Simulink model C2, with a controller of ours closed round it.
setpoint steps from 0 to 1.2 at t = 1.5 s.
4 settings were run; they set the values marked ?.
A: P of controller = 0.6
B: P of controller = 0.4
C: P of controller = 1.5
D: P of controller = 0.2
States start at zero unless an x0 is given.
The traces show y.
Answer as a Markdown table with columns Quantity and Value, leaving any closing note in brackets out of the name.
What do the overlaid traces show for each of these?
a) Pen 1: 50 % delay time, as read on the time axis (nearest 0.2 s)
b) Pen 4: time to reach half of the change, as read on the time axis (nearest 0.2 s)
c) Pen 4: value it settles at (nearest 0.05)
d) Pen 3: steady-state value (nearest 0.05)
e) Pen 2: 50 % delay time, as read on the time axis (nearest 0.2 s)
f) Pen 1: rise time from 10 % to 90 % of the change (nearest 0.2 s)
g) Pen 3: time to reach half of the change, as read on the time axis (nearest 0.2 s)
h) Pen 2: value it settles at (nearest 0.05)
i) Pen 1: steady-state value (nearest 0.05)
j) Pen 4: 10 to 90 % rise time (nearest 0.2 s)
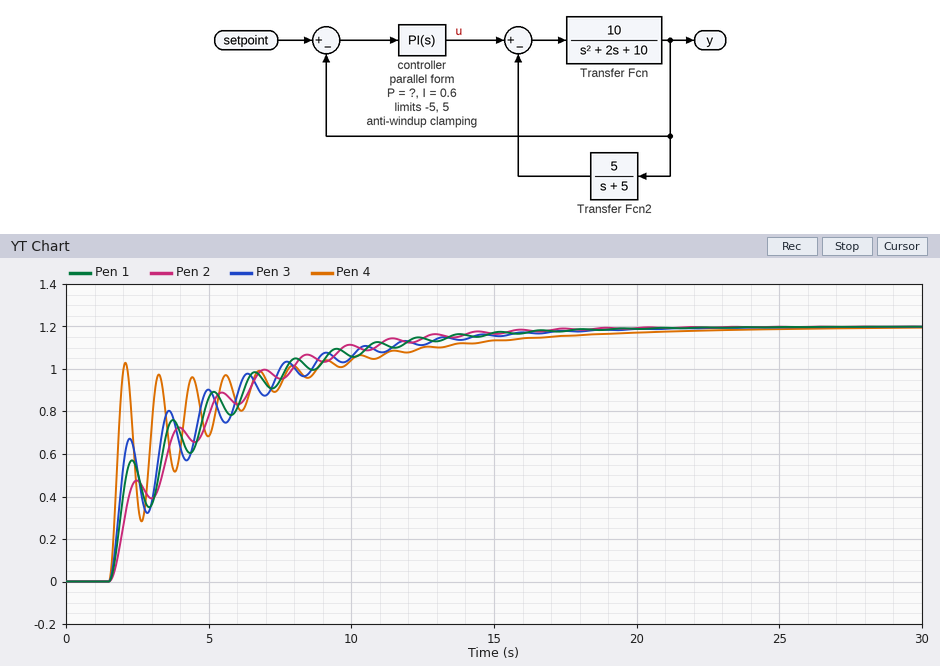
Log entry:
| Quantity | Value |
|---|---|
| Pen 1: 50 % delay time, as read on the time axis | 3.4 s |
| Pen 4: time to reach half of the change, as read on the time axis | 1.8 s |
| Pen 4: value it settles at | 1.20 |
| Pen 3: steady-state value | 1.20 |
| Pen 2: 50 % delay time, as read on the time axis | 3.6 s |
| Pen 1: rise time from 10 % to 90 % of the change | 7.6 s |
| Pen 3: time to reach half of the change, as read on the time axis | 2.0 s |
| Pen 2: value it settles at | 1.20 |
| Pen 1: steady-state value | 1.20 |
| Pen 4: 10 to 90 % rise time | 9.6 s |
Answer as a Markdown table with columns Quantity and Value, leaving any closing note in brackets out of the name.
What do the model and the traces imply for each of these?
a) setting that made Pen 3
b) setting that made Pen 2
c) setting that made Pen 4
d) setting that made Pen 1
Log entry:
| Quantity | Value |
|---|---|
| setting that made Pen 3 | A |
| setting that made Pen 2 | D |
| setting that made Pen 4 | C |
| setting that made Pen 1 | B |
